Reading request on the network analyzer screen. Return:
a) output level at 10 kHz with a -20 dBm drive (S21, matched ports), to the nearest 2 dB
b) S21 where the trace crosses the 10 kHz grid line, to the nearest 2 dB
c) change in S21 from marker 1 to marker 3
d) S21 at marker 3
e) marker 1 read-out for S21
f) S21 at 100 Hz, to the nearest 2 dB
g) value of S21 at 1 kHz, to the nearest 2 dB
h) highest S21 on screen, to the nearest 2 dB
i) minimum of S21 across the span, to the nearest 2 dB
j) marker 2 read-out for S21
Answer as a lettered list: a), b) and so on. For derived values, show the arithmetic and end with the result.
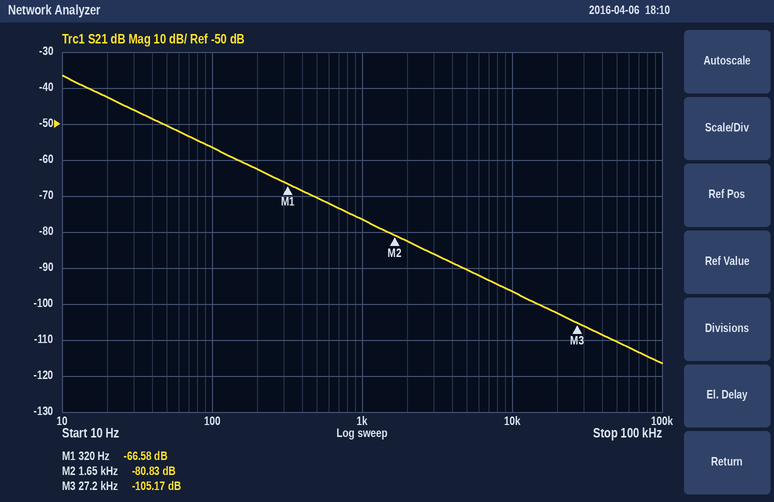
a) -20 dBm + (-96 dB) = -116 dBm
b) -96 dB
c) -105.17 − (-66.58) = -38.59 dB
d) -105.17 dB
e) -66.58 dB
f) -56 dB
g) -76 dB
h) -36 dB
i) -116 dB
j) -80.83 dB
